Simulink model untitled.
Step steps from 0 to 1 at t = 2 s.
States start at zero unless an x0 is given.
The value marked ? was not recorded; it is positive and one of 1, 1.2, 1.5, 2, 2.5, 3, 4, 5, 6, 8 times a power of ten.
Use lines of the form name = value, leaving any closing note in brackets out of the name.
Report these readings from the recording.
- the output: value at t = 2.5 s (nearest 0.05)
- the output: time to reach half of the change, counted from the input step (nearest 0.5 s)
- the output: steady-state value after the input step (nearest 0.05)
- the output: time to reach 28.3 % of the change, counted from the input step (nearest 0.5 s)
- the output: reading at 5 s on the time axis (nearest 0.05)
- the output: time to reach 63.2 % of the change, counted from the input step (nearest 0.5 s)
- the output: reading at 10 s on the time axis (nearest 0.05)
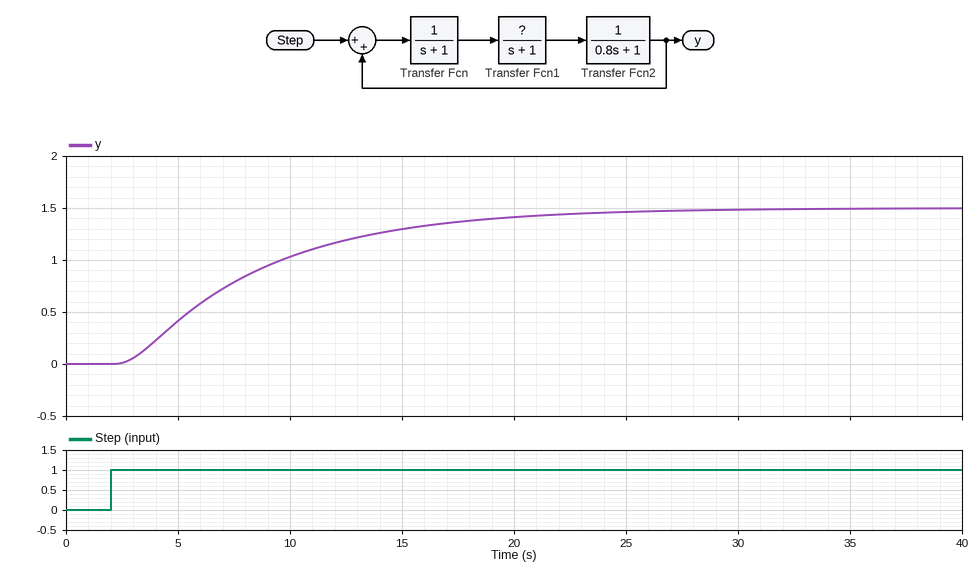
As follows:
the output: value at t = 2.5 s = 0.00
the output: time to reach half of the change, counted from the input step = 5.0 s
the output: steady-state value after the input step = 1.50
the output: time to reach 28.3 % of the change, counted from the input step = 3.0 s
the output: reading at 5 s on the time axis = 0.40
the output: time to reach 63.2 % of the change, counted from the input step = 7.0 s
the output: reading at 10 s on the time axis = 1.05
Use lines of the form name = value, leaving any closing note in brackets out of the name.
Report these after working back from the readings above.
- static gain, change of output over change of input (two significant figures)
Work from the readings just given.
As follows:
static gain, change of output over change of input = 1.5
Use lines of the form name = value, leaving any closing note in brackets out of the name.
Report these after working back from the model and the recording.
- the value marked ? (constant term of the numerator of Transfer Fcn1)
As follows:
the value marked ? = 0.6
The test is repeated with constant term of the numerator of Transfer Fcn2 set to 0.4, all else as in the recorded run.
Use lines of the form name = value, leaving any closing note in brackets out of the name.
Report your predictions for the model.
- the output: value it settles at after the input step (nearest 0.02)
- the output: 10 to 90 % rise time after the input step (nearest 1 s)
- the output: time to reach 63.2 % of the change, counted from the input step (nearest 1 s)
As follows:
the output: value it settles at after the input step = 0.32
the output: 10 to 90 % rise time after the input step = 6 s
the output: time to reach 63.2 % of the change, counted from the input step = 4 s
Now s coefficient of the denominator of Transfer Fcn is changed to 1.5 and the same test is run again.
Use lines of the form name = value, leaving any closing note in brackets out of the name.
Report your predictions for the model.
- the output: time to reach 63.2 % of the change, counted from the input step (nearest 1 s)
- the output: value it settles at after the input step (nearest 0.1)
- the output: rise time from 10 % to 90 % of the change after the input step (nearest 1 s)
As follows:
the output: time to reach 63.2 % of the change, counted from the input step = 8 s
the output: value it settles at after the input step = 1.5
the output: rise time from 10 % to 90 % of the change after the input step = 16 s
